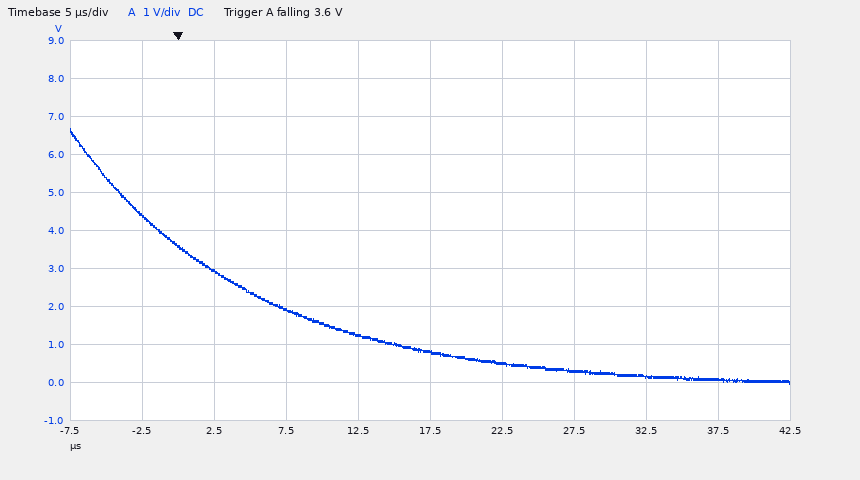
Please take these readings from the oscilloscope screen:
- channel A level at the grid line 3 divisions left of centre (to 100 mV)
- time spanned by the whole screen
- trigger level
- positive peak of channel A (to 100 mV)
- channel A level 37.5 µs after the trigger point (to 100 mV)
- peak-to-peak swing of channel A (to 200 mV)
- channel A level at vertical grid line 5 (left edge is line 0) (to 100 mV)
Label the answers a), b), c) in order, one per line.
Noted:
a) 2.9 V
b) 50 µs
c) 3.6 V
d) 6.7 V
e) 100 mV
f) 6.8 V
g) 800 mV
